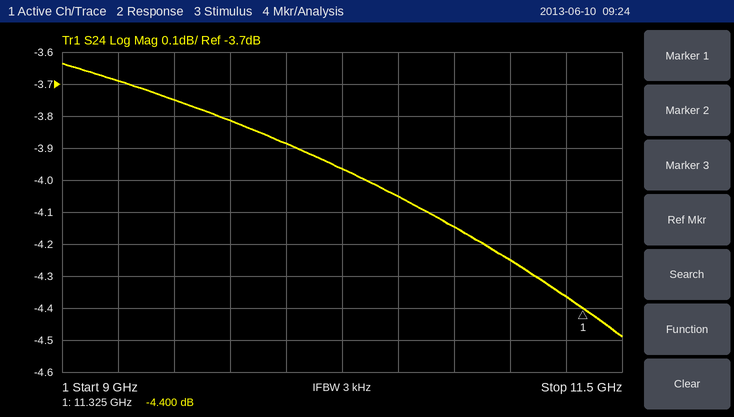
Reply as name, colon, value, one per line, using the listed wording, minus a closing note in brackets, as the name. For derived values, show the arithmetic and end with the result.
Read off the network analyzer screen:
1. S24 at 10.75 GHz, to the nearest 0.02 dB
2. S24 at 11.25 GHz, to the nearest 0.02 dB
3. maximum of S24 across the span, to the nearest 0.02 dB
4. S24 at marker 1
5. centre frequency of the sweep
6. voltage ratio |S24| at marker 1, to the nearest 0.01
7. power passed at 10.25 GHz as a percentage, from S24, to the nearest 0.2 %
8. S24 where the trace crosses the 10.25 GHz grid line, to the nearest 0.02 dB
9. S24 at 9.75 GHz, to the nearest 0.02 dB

S24 at 10.75 GHz, to the nearest 0.02 dB: -4.14 dB
S24 at 11.25 GHz, to the nearest 0.02 dB: -4.36 dB
maximum of S24 across the span, to the nearest 0.02 dB: -3.64 dB
S24 at marker 1: -4.400 dB
centre frequency of the sweep: 10.25 GHz
voltage ratio |S24| at marker 1, to the nearest 0.01: 10^(-4.4/20) ≈ 0.60
power passed at 10.25 GHz as a percentage, from S24, to the nearest 0.2 %: 10^(-3.96/10) ≈ 40.2 %
S24 where the trace crosses the 10.25 GHz grid line, to the nearest 0.02 dB: -3.96 dB
S24 at 9.75 GHz, to the nearest 0.02 dB: -3.82 dB
